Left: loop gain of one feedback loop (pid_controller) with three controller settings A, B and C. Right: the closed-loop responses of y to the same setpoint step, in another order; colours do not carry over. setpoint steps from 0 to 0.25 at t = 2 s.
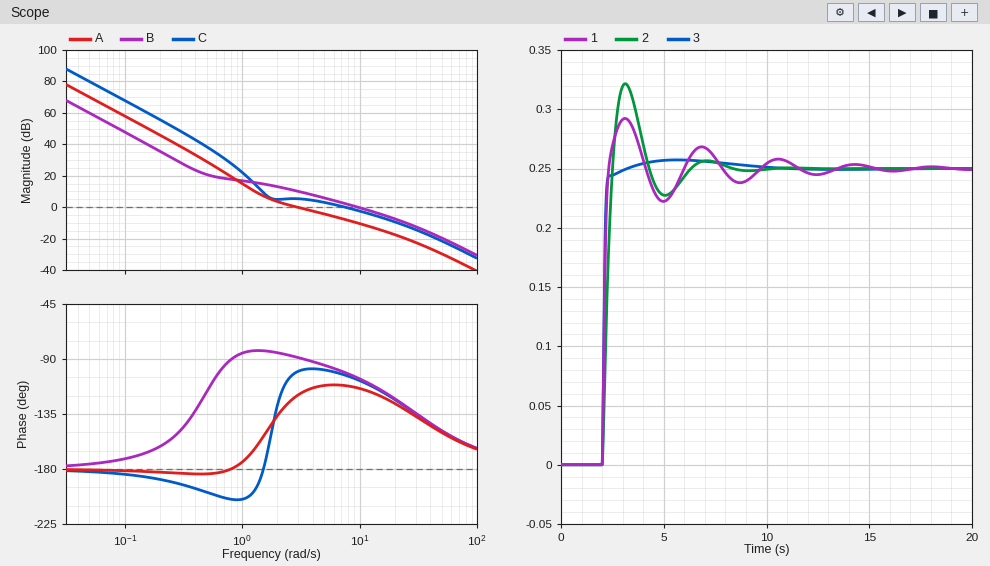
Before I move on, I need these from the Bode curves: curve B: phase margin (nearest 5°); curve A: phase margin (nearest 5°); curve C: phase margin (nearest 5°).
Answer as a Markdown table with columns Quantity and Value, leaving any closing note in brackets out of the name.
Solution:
| Quantity | Value |
|---|---|
| curve B: phase margin | 75° |
| curve A: phase margin | 60° |
| curve C: phase margin | 75° |
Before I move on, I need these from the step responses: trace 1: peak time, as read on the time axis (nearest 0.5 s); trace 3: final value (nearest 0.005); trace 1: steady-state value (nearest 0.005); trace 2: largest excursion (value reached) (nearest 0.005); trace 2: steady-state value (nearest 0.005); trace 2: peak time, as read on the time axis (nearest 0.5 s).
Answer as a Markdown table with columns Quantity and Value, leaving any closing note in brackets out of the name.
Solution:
| Quantity | Value |
|---|---|
| trace 1: peak time, as read on the time axis | 3.0 s |
| trace 3: final value | 0.250 |
| trace 1: steady-state value | 0.250 |
| trace 2: largest excursion (value reached) | 0.320 |
| trace 2: steady-state value | 0.250 |
| trace 2: peak time, as read on the time axis | 3.0 s |
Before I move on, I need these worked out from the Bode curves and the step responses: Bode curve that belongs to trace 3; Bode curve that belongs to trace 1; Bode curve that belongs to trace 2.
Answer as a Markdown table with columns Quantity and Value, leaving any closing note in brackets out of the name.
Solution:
| Quantity | Value |
|---|---|
| Bode curve that belongs to trace 3 | B |
| Bode curve that belongs to trace 1 | C |
| Bode curve that belongs to trace 2 | A |
